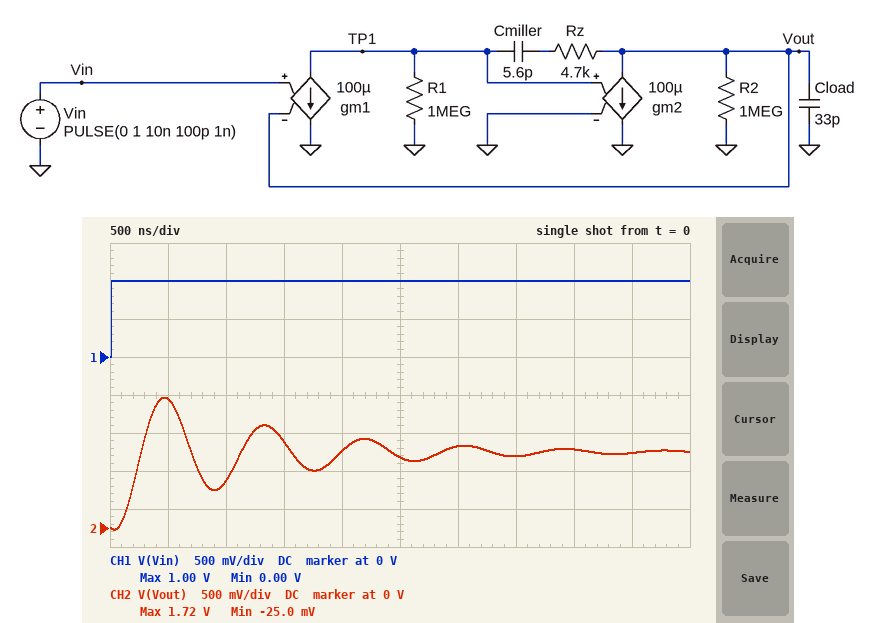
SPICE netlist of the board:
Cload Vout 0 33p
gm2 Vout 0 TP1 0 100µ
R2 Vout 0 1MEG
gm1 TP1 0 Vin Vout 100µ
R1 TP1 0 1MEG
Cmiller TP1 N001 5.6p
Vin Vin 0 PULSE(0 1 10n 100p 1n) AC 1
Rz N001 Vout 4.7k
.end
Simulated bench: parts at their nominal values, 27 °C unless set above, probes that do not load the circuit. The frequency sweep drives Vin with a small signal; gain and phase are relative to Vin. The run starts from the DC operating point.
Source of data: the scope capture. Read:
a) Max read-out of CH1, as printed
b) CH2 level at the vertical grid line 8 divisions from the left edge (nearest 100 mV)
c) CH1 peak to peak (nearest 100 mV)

1.00 V
1.0 V
1.0 V
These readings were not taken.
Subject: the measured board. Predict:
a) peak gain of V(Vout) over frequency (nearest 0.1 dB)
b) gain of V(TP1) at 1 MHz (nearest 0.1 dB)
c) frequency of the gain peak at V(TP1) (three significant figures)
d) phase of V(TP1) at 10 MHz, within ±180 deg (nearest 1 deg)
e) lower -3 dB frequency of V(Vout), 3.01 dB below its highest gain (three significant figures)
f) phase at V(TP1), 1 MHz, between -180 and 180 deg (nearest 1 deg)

13.2 dB
17.4 dB
1.17 MHz
146 deg
1.01 MHz
-118 deg
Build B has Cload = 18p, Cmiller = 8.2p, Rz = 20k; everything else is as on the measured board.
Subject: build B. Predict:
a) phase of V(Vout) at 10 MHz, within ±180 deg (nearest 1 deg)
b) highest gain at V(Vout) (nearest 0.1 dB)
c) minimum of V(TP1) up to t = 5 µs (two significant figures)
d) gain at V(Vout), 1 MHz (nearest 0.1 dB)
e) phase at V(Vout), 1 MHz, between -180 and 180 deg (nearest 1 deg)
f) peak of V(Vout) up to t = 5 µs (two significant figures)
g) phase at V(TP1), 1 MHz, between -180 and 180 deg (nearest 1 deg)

-91 deg
0.3 dB
-2.0 V
0 dB
-42 deg
1.1 V
-124 deg
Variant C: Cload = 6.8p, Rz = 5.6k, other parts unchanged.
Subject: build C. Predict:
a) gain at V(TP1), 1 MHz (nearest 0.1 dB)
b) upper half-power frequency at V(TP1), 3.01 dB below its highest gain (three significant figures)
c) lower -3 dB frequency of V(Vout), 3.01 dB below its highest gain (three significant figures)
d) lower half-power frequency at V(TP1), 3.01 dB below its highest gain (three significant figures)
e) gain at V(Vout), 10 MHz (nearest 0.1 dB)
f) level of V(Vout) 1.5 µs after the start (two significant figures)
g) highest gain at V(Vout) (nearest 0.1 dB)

-0.9 dB
3.40 MHz
1.58 MHz
1.99 MHz
-17.8 dB
1.0 V
6.3 dB
